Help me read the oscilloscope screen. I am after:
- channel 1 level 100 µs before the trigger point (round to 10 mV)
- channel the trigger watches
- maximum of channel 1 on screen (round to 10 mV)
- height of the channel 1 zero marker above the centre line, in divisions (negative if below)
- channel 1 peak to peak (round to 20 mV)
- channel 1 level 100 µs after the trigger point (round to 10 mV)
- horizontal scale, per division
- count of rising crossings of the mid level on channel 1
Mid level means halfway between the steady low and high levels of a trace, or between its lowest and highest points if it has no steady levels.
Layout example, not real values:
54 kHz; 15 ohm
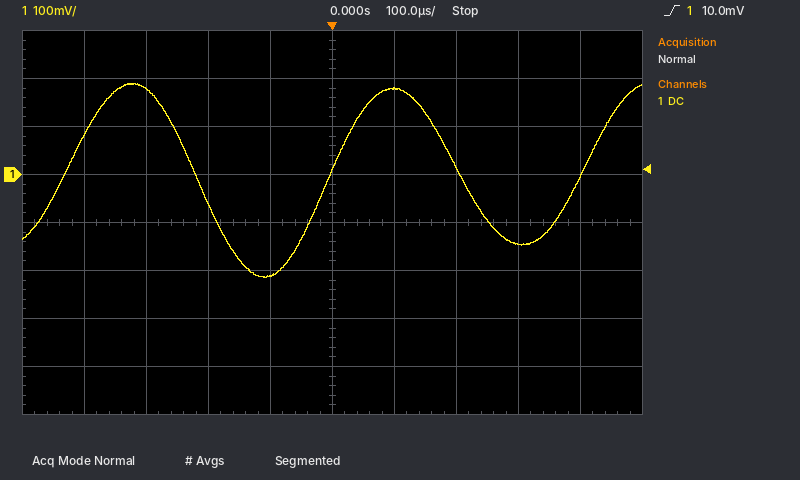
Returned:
-210 mV; channel 1; 190 mV; +1.0 div; 400 mV; 180 mV; 100 µs; 3
